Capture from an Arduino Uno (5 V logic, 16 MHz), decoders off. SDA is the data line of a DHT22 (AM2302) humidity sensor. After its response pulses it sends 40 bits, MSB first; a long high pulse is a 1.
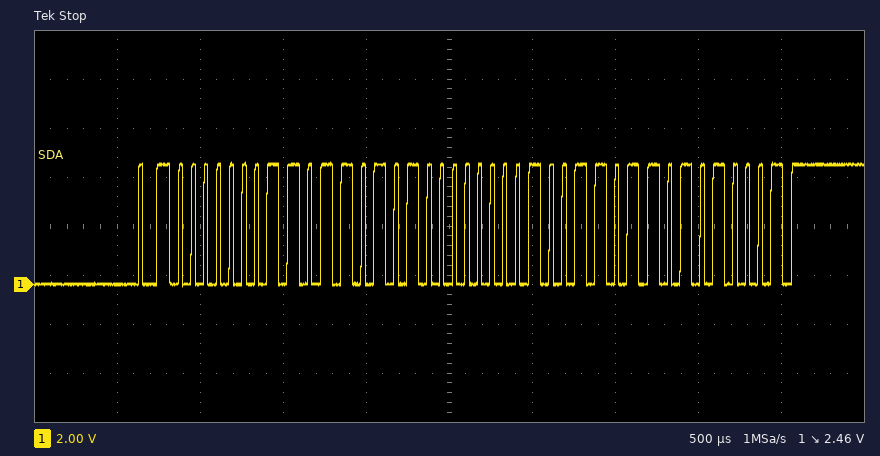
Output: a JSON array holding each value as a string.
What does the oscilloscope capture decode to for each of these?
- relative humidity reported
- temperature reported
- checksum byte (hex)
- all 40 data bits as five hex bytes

["43.7 %", "15.5 °C", "0x51", "01 B5 00 9B 51"]
